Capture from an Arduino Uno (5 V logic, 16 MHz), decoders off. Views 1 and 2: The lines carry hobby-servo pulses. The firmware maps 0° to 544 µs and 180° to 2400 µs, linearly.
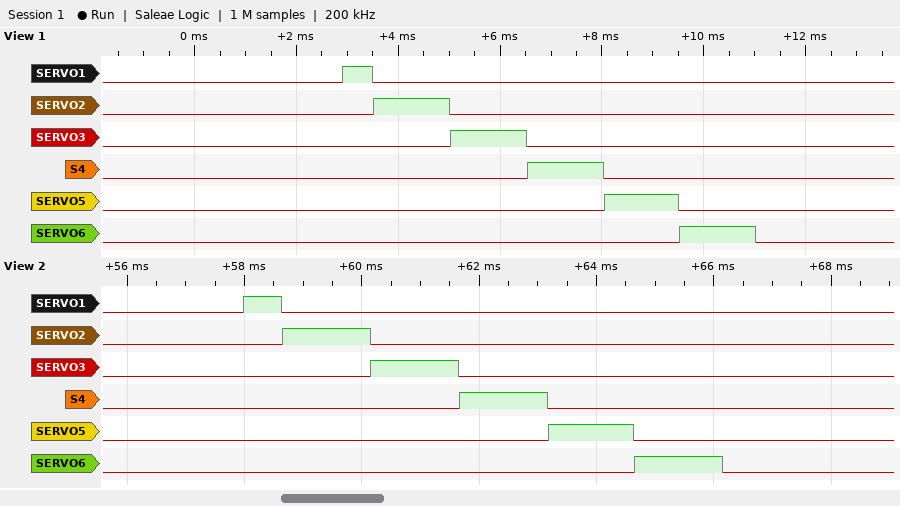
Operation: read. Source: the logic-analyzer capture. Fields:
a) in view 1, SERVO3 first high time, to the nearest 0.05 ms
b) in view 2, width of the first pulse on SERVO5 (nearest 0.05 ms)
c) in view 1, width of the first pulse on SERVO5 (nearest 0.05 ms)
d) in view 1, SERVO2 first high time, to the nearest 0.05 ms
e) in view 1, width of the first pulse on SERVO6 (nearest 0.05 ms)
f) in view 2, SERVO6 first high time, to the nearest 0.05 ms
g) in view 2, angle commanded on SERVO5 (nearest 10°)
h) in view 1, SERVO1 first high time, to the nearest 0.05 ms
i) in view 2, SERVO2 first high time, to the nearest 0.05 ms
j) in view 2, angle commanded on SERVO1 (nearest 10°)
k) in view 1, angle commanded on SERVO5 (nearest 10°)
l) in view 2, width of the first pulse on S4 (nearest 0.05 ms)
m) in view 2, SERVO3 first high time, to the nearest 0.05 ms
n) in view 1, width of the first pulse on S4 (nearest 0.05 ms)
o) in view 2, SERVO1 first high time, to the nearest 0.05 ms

1.50 ms
1.45 ms
1.45 ms
1.50 ms
1.50 ms
1.50 ms
90°
0.60 ms
1.50 ms
10°
90°
1.50 ms
1.50 ms
1.50 ms
0.65 ms
